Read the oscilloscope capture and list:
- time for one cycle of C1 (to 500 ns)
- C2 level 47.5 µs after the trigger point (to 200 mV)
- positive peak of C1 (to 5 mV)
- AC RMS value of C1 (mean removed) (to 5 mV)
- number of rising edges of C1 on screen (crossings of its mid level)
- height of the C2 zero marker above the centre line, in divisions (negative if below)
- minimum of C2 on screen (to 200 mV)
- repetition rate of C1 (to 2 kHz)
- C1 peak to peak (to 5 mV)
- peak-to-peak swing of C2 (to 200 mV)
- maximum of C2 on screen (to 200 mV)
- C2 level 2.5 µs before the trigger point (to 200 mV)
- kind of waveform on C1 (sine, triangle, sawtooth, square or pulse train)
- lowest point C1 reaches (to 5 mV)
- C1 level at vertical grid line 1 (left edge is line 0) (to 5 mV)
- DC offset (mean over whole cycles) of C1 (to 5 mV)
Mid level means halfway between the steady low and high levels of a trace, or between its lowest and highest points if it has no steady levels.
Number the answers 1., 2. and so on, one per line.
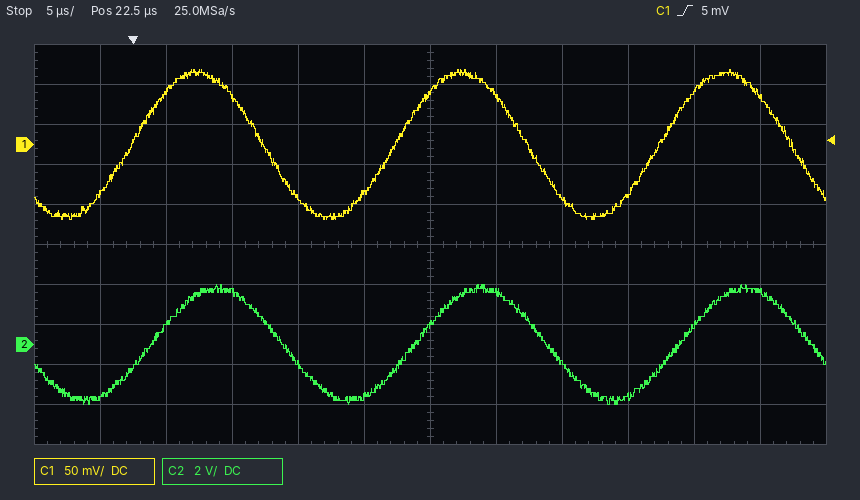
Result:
1. 20.0 µs
2. 2.6 V
3. 95 mV
4. 65 mV
5. 3
6. -2.5 div
7. -3.0 V
8. 50 kHz
9. 190 mV
10. 6.0 V
11. 3.0 V
12. -2.6 V
13. sine
14. -95 mV
15. -60 mV
16. 0 mV
